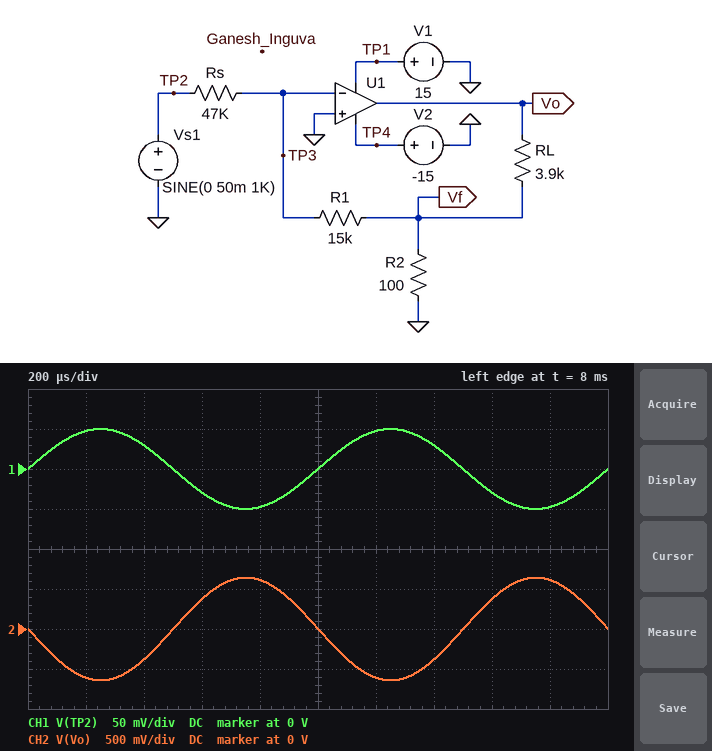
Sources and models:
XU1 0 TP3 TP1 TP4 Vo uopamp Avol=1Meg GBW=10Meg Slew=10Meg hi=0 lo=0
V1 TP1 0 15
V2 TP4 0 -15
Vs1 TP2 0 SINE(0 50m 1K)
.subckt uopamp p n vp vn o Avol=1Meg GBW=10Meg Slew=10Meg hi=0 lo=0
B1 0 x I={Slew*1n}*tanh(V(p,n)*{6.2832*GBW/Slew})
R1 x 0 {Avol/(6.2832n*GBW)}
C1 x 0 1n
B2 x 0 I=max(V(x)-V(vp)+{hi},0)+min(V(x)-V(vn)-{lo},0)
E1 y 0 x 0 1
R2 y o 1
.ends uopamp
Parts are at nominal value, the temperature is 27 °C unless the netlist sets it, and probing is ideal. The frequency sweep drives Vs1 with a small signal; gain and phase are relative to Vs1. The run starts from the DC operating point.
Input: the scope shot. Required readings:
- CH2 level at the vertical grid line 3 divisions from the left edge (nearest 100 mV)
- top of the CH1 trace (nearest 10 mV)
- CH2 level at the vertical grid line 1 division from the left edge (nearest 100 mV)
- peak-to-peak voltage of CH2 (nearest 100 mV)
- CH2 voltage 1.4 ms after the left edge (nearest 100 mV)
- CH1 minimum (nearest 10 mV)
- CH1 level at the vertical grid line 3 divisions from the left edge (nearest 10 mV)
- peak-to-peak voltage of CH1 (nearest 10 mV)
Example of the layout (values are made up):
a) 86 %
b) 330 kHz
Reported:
a) 400 mV
b) 50 mV
c) -600 mV
d) 1.3 V
e) -400 mV
f) -50 mV
g) -30 mV
h) 100 mV
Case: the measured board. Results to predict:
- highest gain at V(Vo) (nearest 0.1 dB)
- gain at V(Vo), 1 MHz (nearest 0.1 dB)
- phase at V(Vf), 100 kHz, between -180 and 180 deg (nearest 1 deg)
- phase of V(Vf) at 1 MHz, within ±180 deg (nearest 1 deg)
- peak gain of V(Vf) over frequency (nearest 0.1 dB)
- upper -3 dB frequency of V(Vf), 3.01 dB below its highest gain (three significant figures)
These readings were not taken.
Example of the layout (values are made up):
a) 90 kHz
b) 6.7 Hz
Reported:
a) 22.2 dB
b) 7.6 dB
c) 152 deg
d) 99 deg
e) -9.9 dB
f) 189 kHz
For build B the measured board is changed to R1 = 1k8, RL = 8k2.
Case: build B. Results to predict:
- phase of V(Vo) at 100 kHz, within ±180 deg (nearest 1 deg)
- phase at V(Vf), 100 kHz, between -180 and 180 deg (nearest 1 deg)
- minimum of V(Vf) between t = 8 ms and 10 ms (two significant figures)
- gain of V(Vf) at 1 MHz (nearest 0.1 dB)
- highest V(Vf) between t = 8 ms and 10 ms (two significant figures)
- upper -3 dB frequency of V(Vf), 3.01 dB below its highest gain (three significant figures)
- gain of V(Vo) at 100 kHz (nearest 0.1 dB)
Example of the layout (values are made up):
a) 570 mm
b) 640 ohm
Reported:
a) 139 deg
b) 137 deg
c) -1.9 mV
d) -46.3 dB
e) 1.9 mV
f) 116 kHz
g) 8.1 dB
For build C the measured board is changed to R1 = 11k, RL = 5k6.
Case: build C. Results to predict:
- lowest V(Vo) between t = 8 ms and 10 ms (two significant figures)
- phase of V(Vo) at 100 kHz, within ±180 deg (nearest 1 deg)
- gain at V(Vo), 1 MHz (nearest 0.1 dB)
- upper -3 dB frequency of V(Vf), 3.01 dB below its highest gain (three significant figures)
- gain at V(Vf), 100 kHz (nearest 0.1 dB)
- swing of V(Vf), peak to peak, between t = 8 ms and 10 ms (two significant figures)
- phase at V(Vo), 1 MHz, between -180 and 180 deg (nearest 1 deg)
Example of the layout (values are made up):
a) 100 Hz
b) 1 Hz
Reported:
a) -670 mV
b) 145 deg
c) 5.5 dB
d) 142 kHz
e) -14.4 dB
f) 23 mV
g) 98 deg
